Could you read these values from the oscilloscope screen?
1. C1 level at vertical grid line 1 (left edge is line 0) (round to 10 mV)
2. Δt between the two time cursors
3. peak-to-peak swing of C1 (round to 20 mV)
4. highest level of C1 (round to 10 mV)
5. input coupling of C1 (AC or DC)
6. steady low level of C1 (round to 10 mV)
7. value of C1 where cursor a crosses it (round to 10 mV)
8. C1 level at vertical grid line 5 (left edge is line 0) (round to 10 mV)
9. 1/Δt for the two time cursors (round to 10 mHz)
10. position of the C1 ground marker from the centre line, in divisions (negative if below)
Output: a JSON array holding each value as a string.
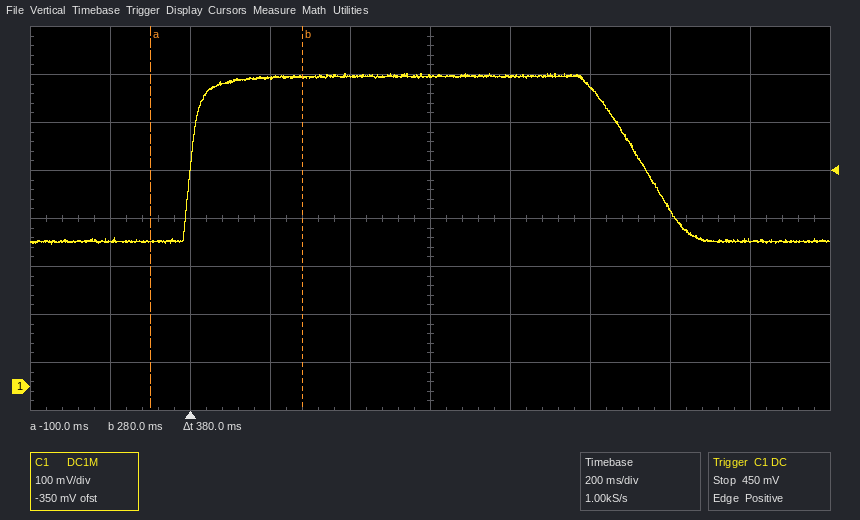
["300 mV", "380 ms", "360 mV", "650 mV", "DC", "300 mV", "300 mV", "650 mV", "2.63 Hz", "-3.5 div"]
